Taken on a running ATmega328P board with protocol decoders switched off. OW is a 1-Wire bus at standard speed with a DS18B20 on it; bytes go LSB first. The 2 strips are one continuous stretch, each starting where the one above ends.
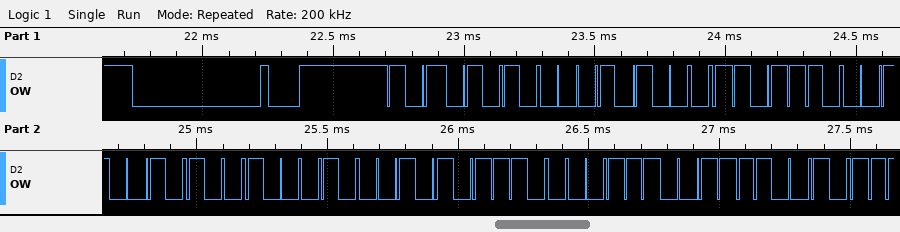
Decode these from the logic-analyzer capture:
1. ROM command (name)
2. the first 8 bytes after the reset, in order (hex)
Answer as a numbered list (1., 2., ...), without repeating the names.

1. Match ROM
2. 55 28 76 A4 44 D4 E1 3C
